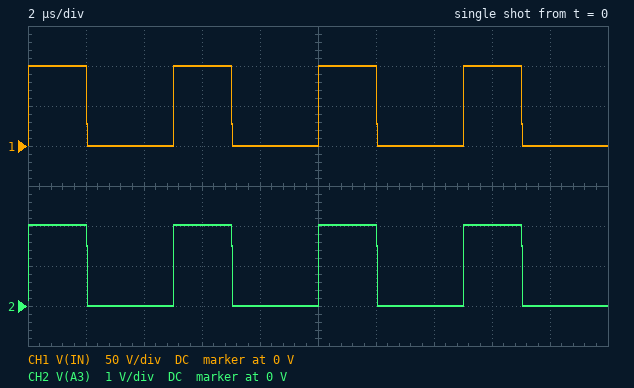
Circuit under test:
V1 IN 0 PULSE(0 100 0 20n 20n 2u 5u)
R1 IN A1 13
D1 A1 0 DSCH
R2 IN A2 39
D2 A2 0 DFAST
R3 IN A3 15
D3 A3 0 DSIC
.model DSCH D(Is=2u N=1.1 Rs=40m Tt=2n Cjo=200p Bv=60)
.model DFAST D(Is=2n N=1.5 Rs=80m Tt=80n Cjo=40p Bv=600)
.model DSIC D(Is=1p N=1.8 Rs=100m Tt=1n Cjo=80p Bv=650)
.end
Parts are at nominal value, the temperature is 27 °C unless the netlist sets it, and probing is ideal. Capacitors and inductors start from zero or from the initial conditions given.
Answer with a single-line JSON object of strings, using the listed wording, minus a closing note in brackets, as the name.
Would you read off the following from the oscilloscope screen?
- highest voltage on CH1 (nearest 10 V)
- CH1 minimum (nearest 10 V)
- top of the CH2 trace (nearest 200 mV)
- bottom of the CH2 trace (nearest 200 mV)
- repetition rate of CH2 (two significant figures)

{"highest voltage on CH1": "100 V", "CH1 minimum": "0 V", "top of the CH2 trace": "2.0 V", "bottom of the CH2 trace": "0 V", "repetition rate of CH2": "200 kHz"}
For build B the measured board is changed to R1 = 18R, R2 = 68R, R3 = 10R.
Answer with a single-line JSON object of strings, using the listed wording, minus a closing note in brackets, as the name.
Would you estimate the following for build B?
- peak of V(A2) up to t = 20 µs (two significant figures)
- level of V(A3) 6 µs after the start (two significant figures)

{"peak of V(A2) up to t = 20 µs": "910 mV", "level of V(A3) 6 µs after the start": "2.4 V"}
